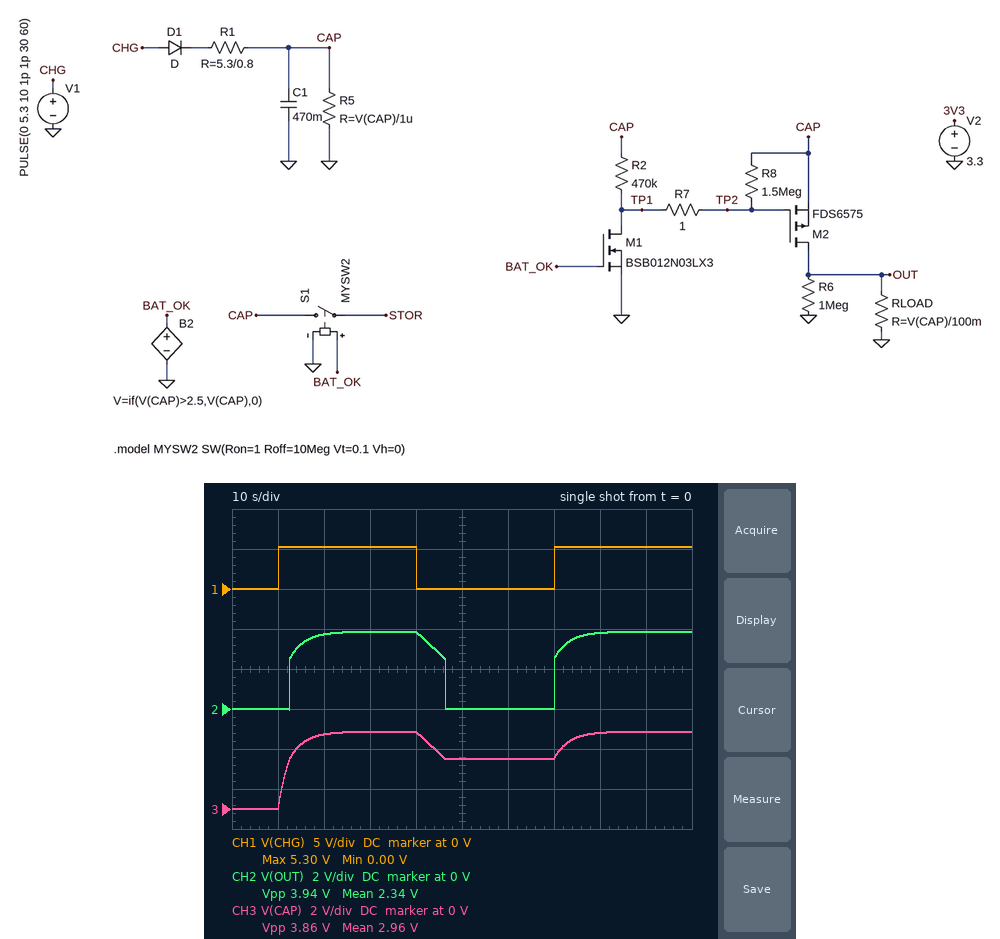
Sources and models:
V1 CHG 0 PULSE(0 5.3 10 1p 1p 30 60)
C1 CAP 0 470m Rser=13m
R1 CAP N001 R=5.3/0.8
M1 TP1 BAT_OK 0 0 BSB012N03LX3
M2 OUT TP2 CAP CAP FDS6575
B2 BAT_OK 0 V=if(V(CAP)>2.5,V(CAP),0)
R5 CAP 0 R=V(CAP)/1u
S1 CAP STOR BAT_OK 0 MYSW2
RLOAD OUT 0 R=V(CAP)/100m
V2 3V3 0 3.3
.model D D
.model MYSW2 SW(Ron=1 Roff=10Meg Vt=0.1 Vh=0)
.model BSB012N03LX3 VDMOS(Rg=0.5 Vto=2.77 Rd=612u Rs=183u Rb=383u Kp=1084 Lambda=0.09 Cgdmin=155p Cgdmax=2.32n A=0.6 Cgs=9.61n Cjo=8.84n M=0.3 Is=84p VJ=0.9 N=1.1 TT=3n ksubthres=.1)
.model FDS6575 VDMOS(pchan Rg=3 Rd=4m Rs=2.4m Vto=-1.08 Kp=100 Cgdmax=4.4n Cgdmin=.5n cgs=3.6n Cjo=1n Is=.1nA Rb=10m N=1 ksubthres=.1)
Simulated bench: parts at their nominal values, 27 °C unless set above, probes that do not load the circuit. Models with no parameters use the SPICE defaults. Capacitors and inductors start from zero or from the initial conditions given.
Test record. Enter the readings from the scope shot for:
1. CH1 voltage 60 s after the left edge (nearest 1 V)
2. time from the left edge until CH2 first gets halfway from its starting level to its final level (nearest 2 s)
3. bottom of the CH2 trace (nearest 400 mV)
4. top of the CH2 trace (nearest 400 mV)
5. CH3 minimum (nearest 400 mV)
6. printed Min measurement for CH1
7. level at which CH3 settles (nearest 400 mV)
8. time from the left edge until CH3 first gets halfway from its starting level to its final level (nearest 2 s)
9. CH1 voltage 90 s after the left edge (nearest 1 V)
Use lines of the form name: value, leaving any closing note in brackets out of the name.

CH1 voltage 60 s after the left edge: 0 V
time from the left edge until CH2 first gets halfway from its starting level to its final level: 12 s
bottom of the CH2 trace: 0 V
top of the CH2 trace: 4.0 V
CH3 minimum: 0 V
printed Min measurement for CH1: 0.00 V
level at which CH3 settles: 4.0 V
time from the left edge until CH3 first gets halfway from its starting level to its final level: 12 s
CH1 voltage 90 s after the left edge: 5 V
